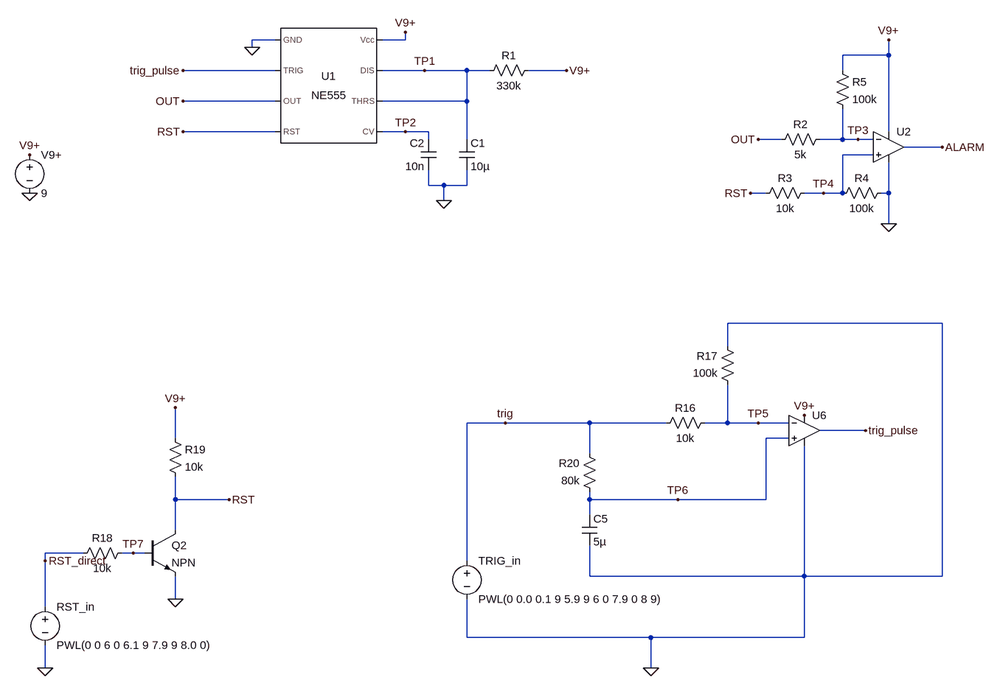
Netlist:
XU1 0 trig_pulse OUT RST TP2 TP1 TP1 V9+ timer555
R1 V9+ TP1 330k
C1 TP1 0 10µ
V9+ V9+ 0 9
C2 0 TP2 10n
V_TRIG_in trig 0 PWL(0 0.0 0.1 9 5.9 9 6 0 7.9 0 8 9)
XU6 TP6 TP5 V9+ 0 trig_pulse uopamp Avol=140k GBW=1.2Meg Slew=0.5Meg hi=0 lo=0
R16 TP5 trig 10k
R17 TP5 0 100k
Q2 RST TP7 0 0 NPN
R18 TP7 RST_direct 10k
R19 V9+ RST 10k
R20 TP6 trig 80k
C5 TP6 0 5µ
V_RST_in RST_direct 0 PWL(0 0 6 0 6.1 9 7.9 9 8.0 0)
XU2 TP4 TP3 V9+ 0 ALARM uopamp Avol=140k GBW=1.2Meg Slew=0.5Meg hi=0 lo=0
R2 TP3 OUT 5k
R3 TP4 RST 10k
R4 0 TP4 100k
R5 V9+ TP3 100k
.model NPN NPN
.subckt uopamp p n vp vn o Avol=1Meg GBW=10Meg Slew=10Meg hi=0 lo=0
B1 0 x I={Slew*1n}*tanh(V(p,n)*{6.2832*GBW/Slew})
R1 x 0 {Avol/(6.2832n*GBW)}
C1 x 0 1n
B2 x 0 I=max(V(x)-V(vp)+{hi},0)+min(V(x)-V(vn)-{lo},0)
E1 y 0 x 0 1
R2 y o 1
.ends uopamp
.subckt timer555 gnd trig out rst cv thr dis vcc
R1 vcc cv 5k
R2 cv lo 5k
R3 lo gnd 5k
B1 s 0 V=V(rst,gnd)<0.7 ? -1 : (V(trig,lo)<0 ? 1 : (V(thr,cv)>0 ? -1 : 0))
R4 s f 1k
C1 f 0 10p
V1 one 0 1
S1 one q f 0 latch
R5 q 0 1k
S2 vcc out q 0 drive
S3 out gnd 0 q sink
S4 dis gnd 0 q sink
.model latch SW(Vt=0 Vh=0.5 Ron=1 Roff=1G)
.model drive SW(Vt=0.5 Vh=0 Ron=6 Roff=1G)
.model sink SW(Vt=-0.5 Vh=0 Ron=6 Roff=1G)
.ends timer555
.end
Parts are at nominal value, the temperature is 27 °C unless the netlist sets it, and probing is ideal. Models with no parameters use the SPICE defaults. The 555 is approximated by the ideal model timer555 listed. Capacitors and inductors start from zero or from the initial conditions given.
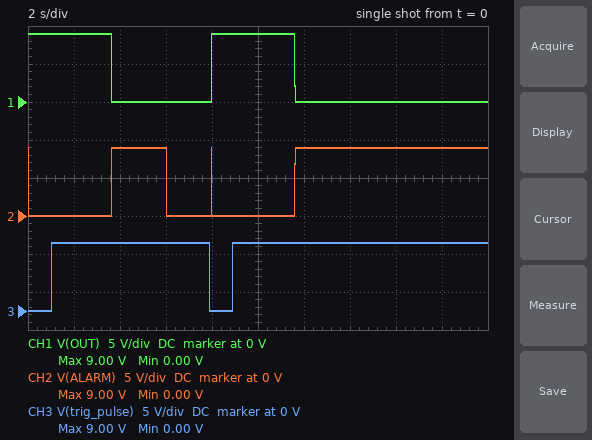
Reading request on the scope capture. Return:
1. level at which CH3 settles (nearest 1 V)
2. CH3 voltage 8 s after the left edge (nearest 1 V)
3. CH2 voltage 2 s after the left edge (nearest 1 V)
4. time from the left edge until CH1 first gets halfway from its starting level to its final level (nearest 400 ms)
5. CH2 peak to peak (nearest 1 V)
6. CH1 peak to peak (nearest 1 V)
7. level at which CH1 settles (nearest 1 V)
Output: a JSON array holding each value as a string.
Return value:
["9 V", "0 V", "0 V", "3.6 s", "9 V", "9 V", "0 V"]
